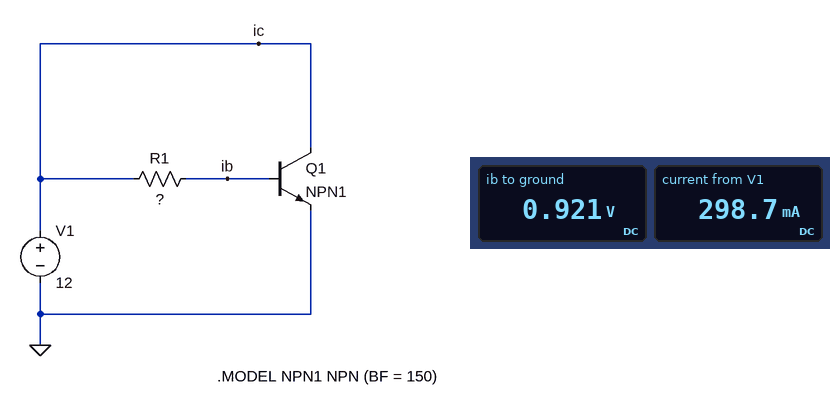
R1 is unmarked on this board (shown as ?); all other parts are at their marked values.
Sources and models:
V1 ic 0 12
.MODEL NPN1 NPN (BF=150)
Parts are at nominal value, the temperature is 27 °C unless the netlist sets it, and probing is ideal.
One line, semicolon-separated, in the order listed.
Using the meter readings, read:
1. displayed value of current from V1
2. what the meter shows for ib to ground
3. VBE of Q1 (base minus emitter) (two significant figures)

298.7 mA; 0.921 V; 920 mV
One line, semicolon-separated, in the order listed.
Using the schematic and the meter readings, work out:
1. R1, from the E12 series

5.6 kΩ
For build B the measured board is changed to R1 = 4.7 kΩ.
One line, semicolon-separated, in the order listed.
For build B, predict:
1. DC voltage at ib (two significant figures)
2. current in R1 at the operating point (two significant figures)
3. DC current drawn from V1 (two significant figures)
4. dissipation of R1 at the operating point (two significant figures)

930 mV; 2.4 mA; 360 mA; 26 mW
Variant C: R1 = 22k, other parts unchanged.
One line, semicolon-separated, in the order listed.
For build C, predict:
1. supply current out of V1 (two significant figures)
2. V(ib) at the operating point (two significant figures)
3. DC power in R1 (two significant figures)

76 mA; 890 mV; 5.6 mW
